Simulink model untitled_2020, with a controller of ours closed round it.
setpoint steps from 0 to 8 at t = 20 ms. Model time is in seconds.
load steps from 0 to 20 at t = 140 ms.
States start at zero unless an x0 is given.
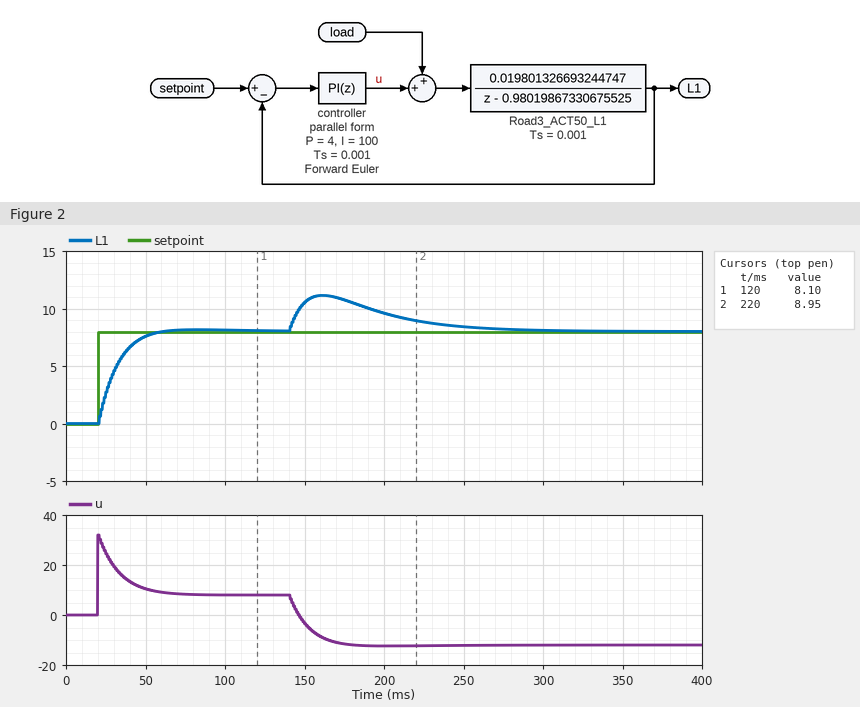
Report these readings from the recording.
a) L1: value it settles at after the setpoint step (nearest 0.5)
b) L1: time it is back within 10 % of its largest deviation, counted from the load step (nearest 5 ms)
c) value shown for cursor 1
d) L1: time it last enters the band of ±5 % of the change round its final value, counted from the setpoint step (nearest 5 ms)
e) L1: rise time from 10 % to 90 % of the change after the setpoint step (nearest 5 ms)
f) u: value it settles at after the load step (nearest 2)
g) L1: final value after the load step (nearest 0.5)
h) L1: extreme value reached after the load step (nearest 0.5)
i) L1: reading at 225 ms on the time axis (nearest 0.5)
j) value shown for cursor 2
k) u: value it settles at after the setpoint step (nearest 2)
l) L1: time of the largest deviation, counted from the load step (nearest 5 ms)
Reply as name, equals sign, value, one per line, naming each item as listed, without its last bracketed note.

L1: value it settles at after the setpoint step = 8.0
L1: time it is back within 10 % of its largest deviation, counted from the load step = 120 ms
value shown for cursor 1 = 8.10
L1: time it last enters the band of ±5 % of the change round its final value, counted from the setpoint step = 30 ms
L1: rise time from 10 % to 90 % of the change after the setpoint step = 25 ms
u: value it settles at after the load step = -12
L1: final value after the load step = 8.0
L1: extreme value reached after the load step = 11.0
L1: reading at 225 ms on the time axis = 9.0
value shown for cursor 2 = 8.95
u: value it settles at after the setpoint step = 8
L1: time of the largest deviation, counted from the load step = 20 ms
